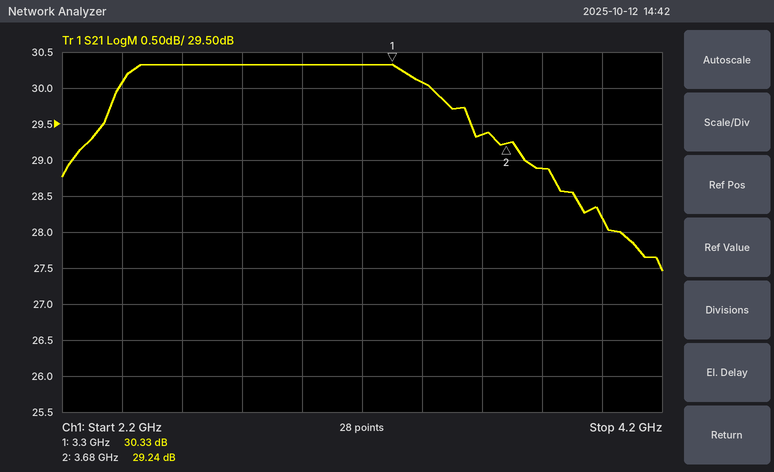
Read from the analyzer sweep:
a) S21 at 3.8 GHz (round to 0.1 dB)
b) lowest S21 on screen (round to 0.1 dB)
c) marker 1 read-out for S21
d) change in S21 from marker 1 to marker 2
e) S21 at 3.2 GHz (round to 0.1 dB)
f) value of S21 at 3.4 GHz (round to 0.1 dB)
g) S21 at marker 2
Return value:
28.9 dB
27.5 dB
30.33 dB
-1.09 dB
30.3 dB
30.1 dB
29.24 dB
